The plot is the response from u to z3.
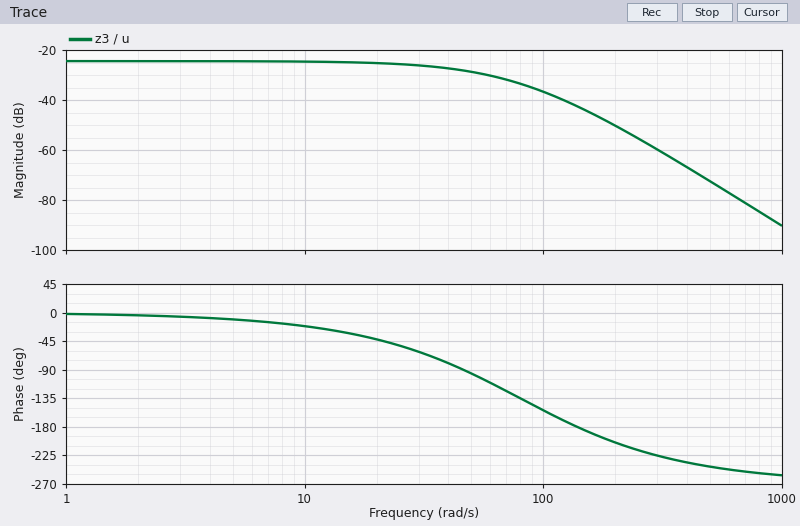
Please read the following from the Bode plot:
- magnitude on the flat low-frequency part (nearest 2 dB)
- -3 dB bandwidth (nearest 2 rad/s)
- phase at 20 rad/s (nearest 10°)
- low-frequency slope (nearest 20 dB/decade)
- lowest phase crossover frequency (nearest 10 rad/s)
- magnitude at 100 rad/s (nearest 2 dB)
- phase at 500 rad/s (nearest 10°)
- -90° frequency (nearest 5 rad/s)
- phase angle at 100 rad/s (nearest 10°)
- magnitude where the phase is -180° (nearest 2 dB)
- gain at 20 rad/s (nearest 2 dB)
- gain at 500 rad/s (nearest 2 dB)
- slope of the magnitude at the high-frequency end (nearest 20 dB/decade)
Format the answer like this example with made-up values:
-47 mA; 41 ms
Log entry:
-24 dB; 40 rad/s; -40°; 0 dB/decade; 140 rad/s; -36 dB; -240°; 45 rad/s; -150°; -42 dB; -26 dB; -72 dB; -60 dB/decade
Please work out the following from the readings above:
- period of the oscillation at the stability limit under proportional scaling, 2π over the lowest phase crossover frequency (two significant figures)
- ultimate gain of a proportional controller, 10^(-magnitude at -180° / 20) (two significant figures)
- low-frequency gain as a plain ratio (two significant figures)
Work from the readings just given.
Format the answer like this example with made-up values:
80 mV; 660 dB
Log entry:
0.045 s; 130; 0.063
